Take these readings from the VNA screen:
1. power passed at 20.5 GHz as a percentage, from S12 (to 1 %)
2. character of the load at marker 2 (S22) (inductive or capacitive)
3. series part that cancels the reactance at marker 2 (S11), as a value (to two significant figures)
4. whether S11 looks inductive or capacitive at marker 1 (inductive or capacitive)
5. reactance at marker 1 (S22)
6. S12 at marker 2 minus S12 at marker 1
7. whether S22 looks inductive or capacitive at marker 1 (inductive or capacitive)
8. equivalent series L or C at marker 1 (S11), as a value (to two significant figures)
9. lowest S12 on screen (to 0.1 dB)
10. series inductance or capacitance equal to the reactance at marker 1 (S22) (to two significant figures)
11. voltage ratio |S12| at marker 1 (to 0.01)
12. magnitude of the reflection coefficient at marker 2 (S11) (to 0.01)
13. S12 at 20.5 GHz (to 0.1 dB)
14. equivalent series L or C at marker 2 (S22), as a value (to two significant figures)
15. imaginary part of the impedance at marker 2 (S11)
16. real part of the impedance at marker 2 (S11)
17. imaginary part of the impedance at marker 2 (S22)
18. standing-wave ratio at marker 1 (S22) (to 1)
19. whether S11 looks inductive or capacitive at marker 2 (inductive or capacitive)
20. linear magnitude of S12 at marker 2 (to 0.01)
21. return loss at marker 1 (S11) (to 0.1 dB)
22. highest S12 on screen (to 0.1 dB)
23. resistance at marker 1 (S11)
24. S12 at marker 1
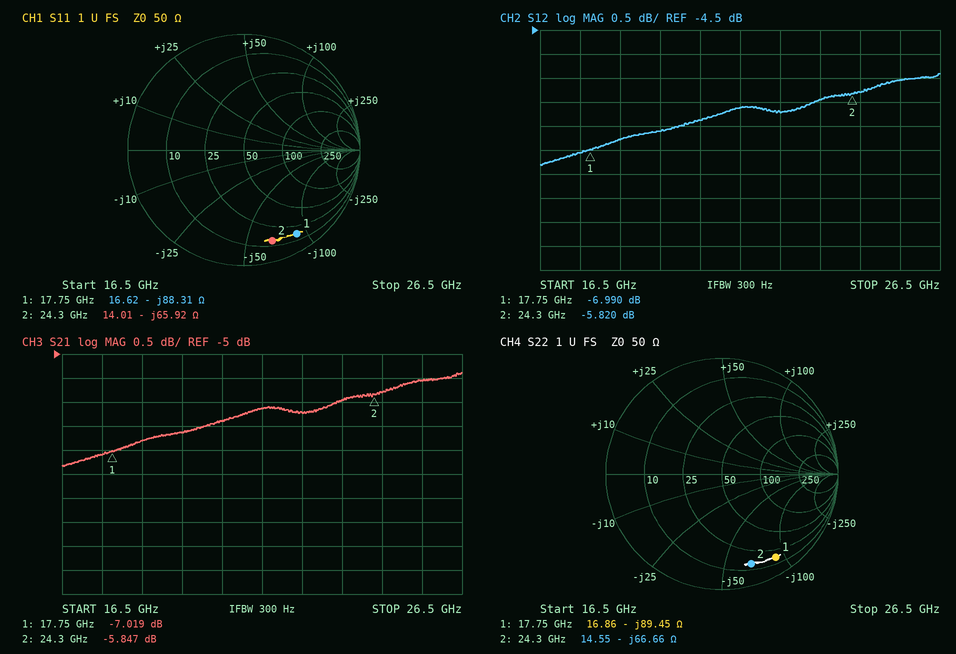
23 %
capacitive
430 pH
capacitive
-89.45 Ω
1.170 dB
capacitive
100 fF
-7.3 dB
100 fF
0.45
0.82
-6.4 dB
98 fF
-65.92 Ω
14.01 Ω
-66.66 Ω
13
capacitive
0.51
1.4 dB
-5.4 dB
16.62 Ω
-6.990 dB
